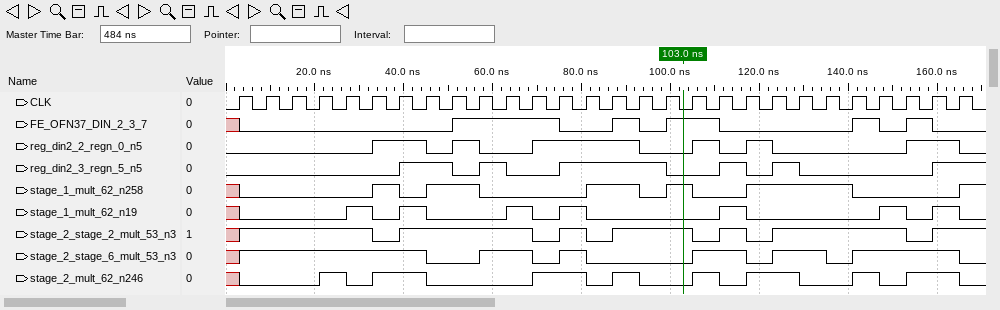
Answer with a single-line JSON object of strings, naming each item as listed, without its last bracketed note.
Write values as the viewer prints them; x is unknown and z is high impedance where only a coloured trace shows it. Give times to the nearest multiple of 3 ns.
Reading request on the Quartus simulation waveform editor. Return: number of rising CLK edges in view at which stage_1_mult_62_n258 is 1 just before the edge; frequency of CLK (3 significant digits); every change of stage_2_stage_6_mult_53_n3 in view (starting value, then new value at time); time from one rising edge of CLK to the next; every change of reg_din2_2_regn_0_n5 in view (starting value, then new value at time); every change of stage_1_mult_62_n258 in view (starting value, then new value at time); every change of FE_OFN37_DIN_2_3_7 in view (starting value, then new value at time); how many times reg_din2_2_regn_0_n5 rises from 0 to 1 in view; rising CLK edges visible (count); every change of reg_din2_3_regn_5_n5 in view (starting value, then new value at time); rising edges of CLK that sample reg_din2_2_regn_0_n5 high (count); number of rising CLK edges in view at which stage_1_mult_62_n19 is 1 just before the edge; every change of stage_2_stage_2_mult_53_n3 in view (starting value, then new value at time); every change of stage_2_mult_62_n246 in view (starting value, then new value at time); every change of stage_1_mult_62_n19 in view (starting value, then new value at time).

{"number of rising CLK edges in view at which stage_1_mult_62_n258 is 1 just before the edge": "10", "frequency of CLK": "167 MHz", "every change of stage_2_stage_6_mult_53_n3 in view": "x, 1 at 3 ns, 0 at 45 ns, 1 at 57 ns, 0 at 69 ns, 1 at 75 ns, 0 at 81 ns, 1 at 105 ns, 0 at 117 ns, 1 at 123 ns, 0 at 135 ns, 1 at 141 ns, 0 at 165 ns", "time from one rising edge of CLK to the next": "6 ns", "every change of reg_din2_2_regn_0_n5 in view": "0, 1 at 33 ns, 0 at 45 ns, 1 at 51 ns, 0 at 57 ns, 1 at 69 ns, 0 at 93 ns, 1 at 105 ns, 0 at 111 ns, 1 at 117 ns, 0 at 123 ns, 1 at 153 ns, 0 at 165 ns", "every change of stage_1_mult_62_n258 in view": "x, 0 at 3 ns, 1 at 33 ns, 0 at 39 ns, 1 at 45 ns, 0 at 57 ns, 1 at 81 ns, 0 at 93 ns, 1 at 99 ns, 0 at 105 ns, 1 at 117 ns, 0 at 141 ns, 1 at 165 ns", "every change of FE_OFN37_DIN_2_3_7 in view": "x, 0 at 3 ns, 1 at 51 ns, 0 at 75 ns, 1 at 87 ns, 0 at 93 ns, 1 at 99 ns, 0 at 111 ns, 1 at 141 ns, 0 at 147 ns, 1 at 153 ns, 0 at 159 ns", "how many times reg_din2_2_regn_0_n5 rises from 0 to 1 in view": "6", "rising CLK edges visible": "28", "every change of reg_din2_3_regn_5_n5 in view": "0, 1 at 39 ns, 0 at 51 ns, 1 at 57 ns, 0 at 63 ns, 1 at 75 ns, 0 at 99 ns, 1 at 111 ns, 0 at 117 ns, 1 at 123 ns, 0 at 129 ns, 1 at 159 ns", "rising edges of CLK that sample reg_din2_2_regn_0_n5 high": "11", "number of rising CLK edges in view at which stage_1_mult_62_n19 is 1 just before the edge": "7", "every change of stage_2_stage_2_mult_53_n3 in view": "x, 1 at 3 ns, 0 at 33 ns, 1 at 39 ns, 0 at 69 ns, 1 at 75 ns, 0 at 81 ns, 1 at 87 ns, 0 at 105 ns, 1 at 111 ns, 0 at 117 ns, 1 at 123 ns, 0 at 153 ns, 1 at 159 ns", "every change of stage_2_mult_62_n246 in view": "x, 0 at 3 ns, 1 at 21 ns, 0 at 27 ns, 1 at 33 ns, 0 at 45 ns, 1 at 69 ns, 0 at 81 ns, 1 at 87 ns, 0 at 93 ns, 1 at 105 ns, 0 at 111 ns, 1 at 117 ns, 0 at 129 ns, 1 at 141 ns, 0 at 147 ns, 1 at 153 ns, 0 at 165 ns", "every change of stage_1_mult_62_n19 in view": "x, 0 at 3 ns, 1 at 27 ns, 0 at 33 ns, 1 at 39 ns, 0 at 45 ns, 1 at 63 ns, 0 at 69 ns, 1 at 75 ns, 0 at 81 ns, 1 at 111 ns, 0 at 117 ns, 1 at 147 ns, 0 at 153 ns, 1 at 159 ns, 0 at 165 ns"}
